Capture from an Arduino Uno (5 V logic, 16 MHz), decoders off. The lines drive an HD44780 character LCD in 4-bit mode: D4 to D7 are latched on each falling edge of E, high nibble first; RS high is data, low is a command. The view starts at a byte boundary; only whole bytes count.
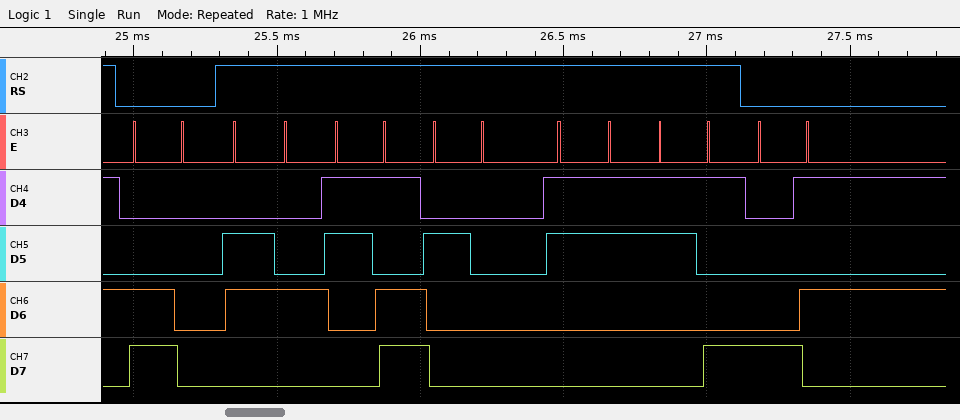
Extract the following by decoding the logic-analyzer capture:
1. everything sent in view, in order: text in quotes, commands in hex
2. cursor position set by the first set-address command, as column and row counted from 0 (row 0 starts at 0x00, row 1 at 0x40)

0xC0 "d= 39" 0x85
column 0, row 1
